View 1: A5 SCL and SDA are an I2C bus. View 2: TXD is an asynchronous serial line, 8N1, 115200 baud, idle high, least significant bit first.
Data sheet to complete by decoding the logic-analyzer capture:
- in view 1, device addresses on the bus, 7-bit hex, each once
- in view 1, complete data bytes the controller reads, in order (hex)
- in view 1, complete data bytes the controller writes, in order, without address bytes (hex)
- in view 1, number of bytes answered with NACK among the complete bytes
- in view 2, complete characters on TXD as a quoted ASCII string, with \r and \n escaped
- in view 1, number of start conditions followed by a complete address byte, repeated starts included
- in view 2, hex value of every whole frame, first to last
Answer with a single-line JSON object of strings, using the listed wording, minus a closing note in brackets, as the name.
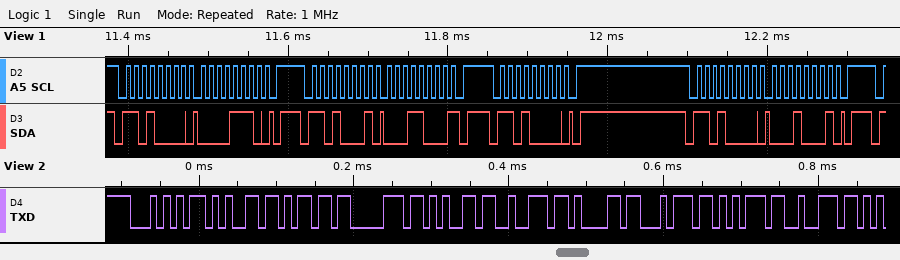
{"in view 1, device addresses on the bus, 7-bit hex, each once": "0x68", "in view 1, complete data bytes the controller reads, in order": "18", "in view 1, complete data bytes the controller writes, in order, without address bytes": "0E 11", "in view 1, number of bytes answered with NACK among the complete bytes": "1", "in view 2, complete characters on TXD as a quoted ASCII string, with \\r and \\n escaped": "\"Temperatur\"", "in view 1, number of start conditions followed by a complete address byte, repeated starts included": "4", "in view 2, hex value of every whole frame, first to last": "54 65 6D 70 65 72 61 74 75 72"}
